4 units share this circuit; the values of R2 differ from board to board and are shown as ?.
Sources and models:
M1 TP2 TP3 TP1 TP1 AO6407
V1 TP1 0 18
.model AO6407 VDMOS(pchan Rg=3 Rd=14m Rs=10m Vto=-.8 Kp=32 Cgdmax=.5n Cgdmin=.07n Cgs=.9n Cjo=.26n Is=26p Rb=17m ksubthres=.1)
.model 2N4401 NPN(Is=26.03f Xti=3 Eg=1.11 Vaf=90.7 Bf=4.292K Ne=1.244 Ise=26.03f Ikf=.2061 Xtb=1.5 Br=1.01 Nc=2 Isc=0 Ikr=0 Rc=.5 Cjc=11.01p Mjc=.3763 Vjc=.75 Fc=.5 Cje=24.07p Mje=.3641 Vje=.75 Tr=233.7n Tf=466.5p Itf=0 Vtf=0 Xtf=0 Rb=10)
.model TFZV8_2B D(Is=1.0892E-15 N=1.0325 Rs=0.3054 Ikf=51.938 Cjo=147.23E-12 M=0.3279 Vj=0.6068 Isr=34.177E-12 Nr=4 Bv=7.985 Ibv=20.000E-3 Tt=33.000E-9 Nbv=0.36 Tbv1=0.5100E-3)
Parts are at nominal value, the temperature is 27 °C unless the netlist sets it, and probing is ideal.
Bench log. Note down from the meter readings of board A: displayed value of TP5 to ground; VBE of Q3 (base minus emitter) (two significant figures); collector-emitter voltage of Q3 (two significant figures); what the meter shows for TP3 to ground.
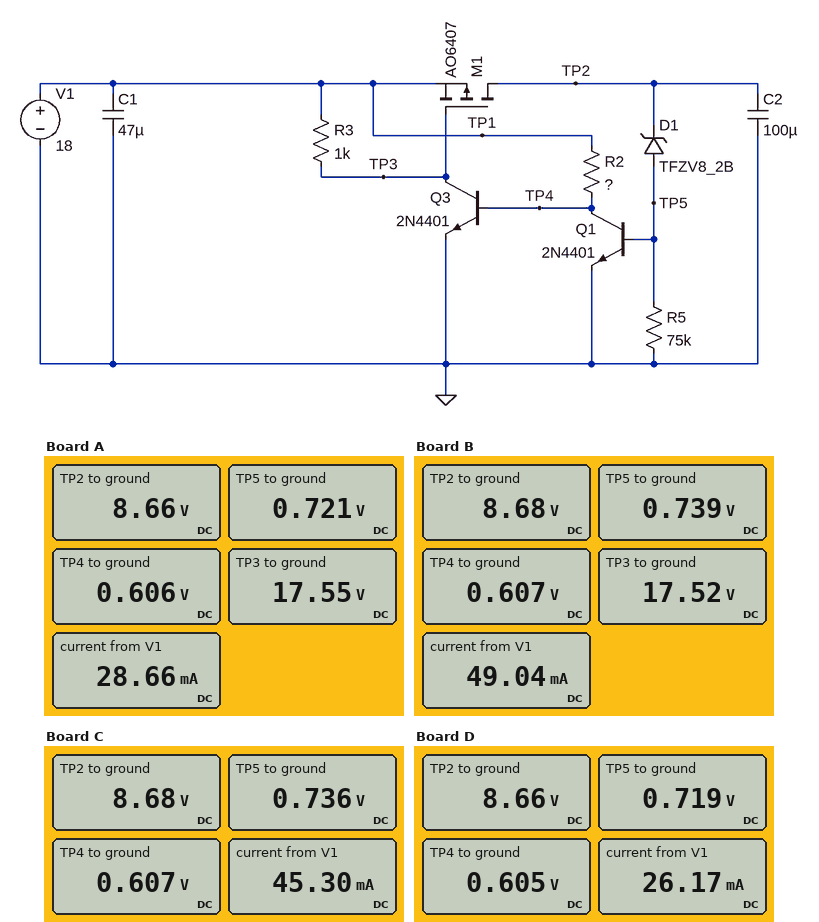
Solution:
0.721 V
610 mV
18 V
17.55 V
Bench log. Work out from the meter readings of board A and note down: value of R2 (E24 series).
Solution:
620 Ω
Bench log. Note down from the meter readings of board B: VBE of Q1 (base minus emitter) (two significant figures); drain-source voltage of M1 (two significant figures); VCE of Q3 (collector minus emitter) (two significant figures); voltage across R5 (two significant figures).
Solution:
740 mV
-9.3 V
18 V
740 mV
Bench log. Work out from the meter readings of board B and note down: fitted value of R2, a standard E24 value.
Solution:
360 Ω
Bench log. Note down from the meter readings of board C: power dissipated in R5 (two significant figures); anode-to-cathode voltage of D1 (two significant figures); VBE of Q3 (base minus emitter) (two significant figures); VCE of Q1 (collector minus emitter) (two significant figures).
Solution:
7.2 µW
-7.9 V
610 mV
610 mV
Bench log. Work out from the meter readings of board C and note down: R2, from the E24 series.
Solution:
390 Ω
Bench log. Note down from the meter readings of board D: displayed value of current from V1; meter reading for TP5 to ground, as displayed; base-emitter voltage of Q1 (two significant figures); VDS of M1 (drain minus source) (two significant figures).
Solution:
26.17 mA
0.719 V
720 mV
-9.3 V
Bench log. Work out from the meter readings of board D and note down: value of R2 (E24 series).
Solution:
680 Ω
